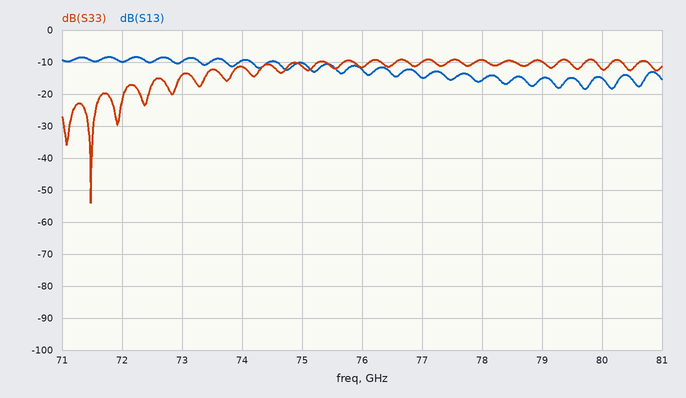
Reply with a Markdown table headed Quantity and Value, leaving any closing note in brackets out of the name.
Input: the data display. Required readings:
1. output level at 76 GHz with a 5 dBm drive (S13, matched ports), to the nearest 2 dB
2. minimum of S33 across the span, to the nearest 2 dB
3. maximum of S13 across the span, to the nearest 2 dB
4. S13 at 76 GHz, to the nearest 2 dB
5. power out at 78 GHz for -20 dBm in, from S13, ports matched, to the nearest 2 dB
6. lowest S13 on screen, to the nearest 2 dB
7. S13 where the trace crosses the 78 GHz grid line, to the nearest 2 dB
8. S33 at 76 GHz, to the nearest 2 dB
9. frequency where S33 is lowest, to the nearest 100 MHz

| Quantity | Value |
|---|---|
| output level at 76 GHz with a 5 dBm drive (S13, matched ports), to the nearest 2 dB | -8 dBm |
| minimum of S33 across the span, to the nearest 2 dB | -54 dB |
| maximum of S13 across the span, to the nearest 2 dB | -8 dB |
| S13 at 76 GHz, to the nearest 2 dB | -12 dB |
| power out at 78 GHz for -20 dBm in, from S13, ports matched, to the nearest 2 dB | -36 dBm |
| lowest S13 on screen, to the nearest 2 dB | -18 dB |
| S13 where the trace crosses the 78 GHz grid line, to the nearest 2 dB | -16 dB |
| S33 at 76 GHz, to the nearest 2 dB | -12 dB |
| frequency where S33 is lowest, to the nearest 100 MHz | 71.5 GHz |
